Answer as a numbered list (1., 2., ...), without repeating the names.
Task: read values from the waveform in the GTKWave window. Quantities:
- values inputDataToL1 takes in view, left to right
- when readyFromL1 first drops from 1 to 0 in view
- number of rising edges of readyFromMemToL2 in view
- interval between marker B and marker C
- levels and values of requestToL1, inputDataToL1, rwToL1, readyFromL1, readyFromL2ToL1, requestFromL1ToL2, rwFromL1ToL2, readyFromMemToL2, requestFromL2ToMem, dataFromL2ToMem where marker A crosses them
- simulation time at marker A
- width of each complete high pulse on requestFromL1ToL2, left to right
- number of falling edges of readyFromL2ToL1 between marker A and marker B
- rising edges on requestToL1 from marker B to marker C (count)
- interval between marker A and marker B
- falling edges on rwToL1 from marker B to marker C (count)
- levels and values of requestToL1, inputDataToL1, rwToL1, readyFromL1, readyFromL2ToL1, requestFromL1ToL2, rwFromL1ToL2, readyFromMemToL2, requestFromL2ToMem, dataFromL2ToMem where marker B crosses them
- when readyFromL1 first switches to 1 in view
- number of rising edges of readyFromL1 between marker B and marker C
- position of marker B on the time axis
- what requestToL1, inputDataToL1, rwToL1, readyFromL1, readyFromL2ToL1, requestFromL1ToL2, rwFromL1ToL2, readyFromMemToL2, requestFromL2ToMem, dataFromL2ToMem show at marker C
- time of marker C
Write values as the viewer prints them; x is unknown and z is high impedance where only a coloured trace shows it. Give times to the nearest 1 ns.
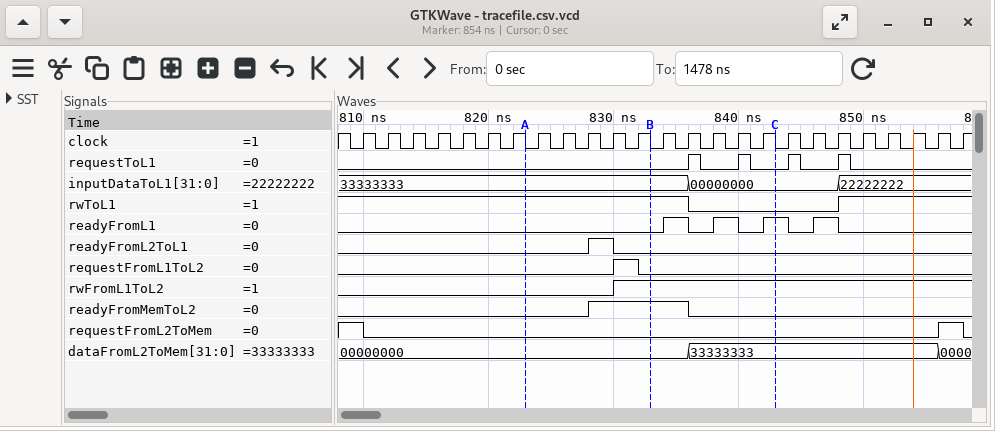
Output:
1. 33333333, 00000000, 22222222
2. 836 ns
3. 1
4. 10 ns
5. requestToL1=0, inputDataToL1=33333333, rwToL1=1, readyFromL1=0, readyFromL2ToL1=0, requestFromL1ToL2=0, rwFromL1ToL2=0, readyFromMemToL2=0, requestFromL2ToMem=0, dataFromL2ToMem=00000000
6. 823 ns
7. 2 ns
8. 1
9. 2
10. 10 ns
11. 1
12. requestToL1=0, inputDataToL1=33333333, rwToL1=1, readyFromL1=0, readyFromL2ToL1=0, requestFromL1ToL2=0, rwFromL1ToL2=1, readyFromMemToL2=1, requestFromL2ToMem=0, dataFromL2ToMem=00000000
13. 834 ns
14. 3
15. 833 ns
16. requestToL1=0, inputDataToL1=00000000, rwToL1=0, readyFromL1=1, readyFromL2ToL1=0, requestFromL1ToL2=0, rwFromL1ToL2=1, readyFromMemToL2=0, requestFromL2ToMem=0, dataFromL2ToMem=33333333
17. 843 ns
